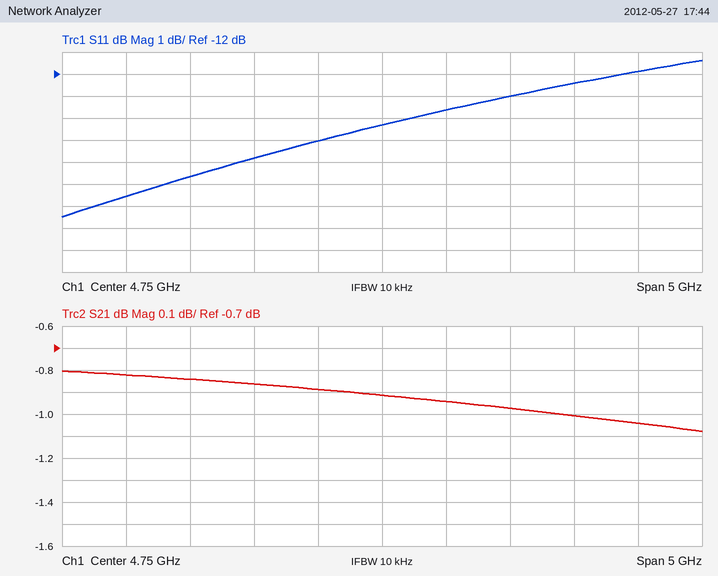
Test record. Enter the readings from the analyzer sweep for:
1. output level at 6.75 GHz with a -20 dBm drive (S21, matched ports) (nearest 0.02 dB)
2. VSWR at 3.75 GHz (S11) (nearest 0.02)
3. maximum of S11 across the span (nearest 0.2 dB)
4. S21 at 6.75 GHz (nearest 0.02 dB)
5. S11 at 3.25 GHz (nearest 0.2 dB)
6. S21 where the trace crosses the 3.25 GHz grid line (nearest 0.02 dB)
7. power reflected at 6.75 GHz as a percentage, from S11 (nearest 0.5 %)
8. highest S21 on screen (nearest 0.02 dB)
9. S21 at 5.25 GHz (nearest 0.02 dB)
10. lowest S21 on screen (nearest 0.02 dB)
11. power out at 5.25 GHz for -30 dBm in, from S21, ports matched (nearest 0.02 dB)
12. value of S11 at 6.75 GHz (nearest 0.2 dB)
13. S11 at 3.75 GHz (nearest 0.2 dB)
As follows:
-21.04 dBm
1.38
-11.4 dB
-1.04 dB
-16.6 dB
-0.84 dB
6.5 %
-0.80 dB
-0.94 dB
-1.08 dB
-30.94 dBm
-11.8 dB
-15.8 dB
